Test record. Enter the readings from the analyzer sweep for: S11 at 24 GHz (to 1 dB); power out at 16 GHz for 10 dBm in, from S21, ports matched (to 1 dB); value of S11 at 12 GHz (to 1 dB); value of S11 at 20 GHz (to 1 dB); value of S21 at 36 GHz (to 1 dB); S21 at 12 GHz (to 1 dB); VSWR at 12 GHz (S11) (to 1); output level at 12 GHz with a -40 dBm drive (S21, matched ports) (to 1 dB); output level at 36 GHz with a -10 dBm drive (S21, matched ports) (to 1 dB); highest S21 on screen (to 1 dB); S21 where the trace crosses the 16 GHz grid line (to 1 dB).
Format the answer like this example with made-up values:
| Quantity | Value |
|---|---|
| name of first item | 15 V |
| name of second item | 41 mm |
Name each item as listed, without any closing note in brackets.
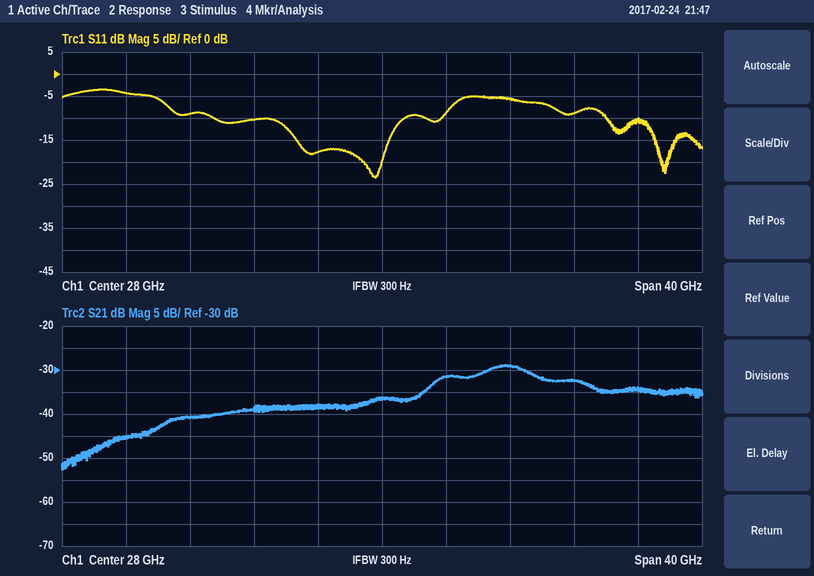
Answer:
| Quantity | Value |
|---|---|
| S11 at 24 GHz | -18 dB |
| power out at 16 GHz for 10 dBm in, from S21, ports matched | -31 dBm |
| value of S11 at 12 GHz | -4 dB |
| value of S11 at 20 GHz | -10 dB |
| value of S21 at 36 GHz | -29 dB |
| S21 at 12 GHz | -45 dB |
| VSWR at 12 GHz (S11) | 4 |
| output level at 12 GHz with a -40 dBm drive (S21, matched ports) | -85 dBm |
| output level at 36 GHz with a -10 dBm drive (S21, matched ports) | -39 dBm |
| highest S21 on screen | -29 dB |
| S21 where the trace crosses the 16 GHz grid line | -41 dB |
